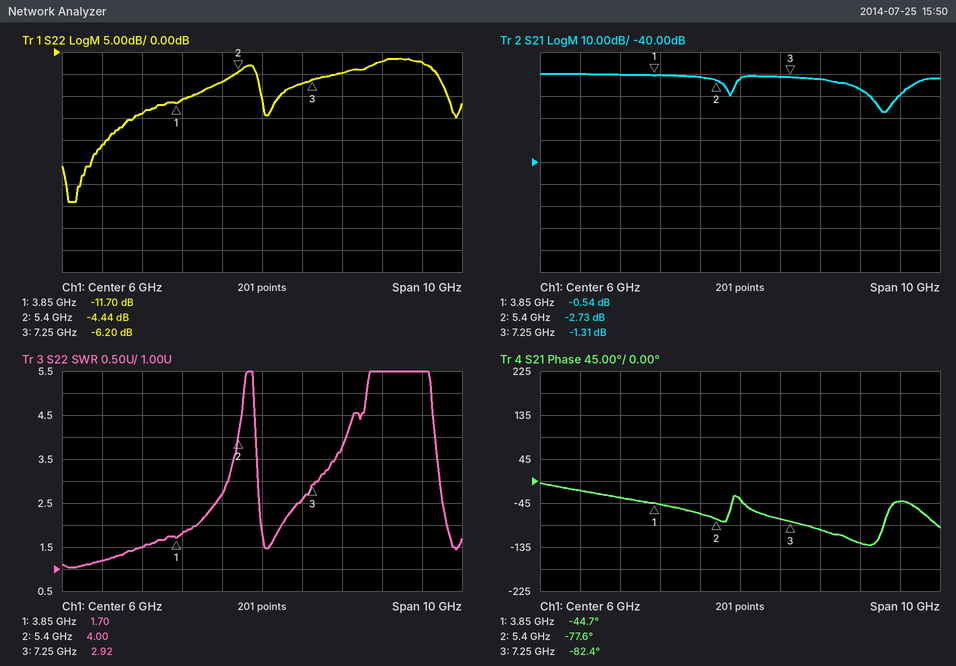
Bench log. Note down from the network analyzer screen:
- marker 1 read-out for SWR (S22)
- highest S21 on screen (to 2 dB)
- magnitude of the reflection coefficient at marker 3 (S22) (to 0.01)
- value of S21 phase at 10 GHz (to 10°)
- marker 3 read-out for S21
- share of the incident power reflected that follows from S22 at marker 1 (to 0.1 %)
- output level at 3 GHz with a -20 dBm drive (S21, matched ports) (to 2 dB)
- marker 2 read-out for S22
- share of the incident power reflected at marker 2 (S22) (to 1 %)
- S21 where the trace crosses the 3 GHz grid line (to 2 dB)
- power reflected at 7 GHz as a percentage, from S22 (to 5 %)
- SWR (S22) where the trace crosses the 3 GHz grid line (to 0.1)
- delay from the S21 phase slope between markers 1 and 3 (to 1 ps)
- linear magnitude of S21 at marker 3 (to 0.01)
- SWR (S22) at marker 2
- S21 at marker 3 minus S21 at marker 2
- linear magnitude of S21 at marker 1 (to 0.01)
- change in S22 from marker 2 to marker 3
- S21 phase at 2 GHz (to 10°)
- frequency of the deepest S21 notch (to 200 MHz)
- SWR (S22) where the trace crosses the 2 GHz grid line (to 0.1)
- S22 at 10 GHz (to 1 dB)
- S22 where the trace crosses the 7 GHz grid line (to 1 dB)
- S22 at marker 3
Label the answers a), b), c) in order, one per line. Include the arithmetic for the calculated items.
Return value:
a) 1.70
b) 0 dB
c) 10^(-6.2/20) ≈ 0.49
d) -40°
e) -1.31 dB
f) 10^(-11.7/10) ≈ 6.8 %
g) -20 dBm + (0 dB) = -20 dBm
h) -4.44 dB
i) 10^(-4.44/10) ≈ 36 %
j) 0 dB
k) 10^(-7/10) ≈ 20 %
l) 1.5
m) −(-82.4° − (-44.7°))/(360° × 3.4 GHz) ≈ 31 ps
n) 10^(-1.31/20) ≈ 0.86
o) 4.00
p) -1.31 − (-2.73) = 1.42 dB
q) 10^(-0.54/20) ≈ 0.94
r) -6.2 − (-4.44) = -1.76 dB
s) -20°
t) 9.6 GHz
u) 1.2
v) -2 dB
w) -7 dB
x) -6.20 dB
